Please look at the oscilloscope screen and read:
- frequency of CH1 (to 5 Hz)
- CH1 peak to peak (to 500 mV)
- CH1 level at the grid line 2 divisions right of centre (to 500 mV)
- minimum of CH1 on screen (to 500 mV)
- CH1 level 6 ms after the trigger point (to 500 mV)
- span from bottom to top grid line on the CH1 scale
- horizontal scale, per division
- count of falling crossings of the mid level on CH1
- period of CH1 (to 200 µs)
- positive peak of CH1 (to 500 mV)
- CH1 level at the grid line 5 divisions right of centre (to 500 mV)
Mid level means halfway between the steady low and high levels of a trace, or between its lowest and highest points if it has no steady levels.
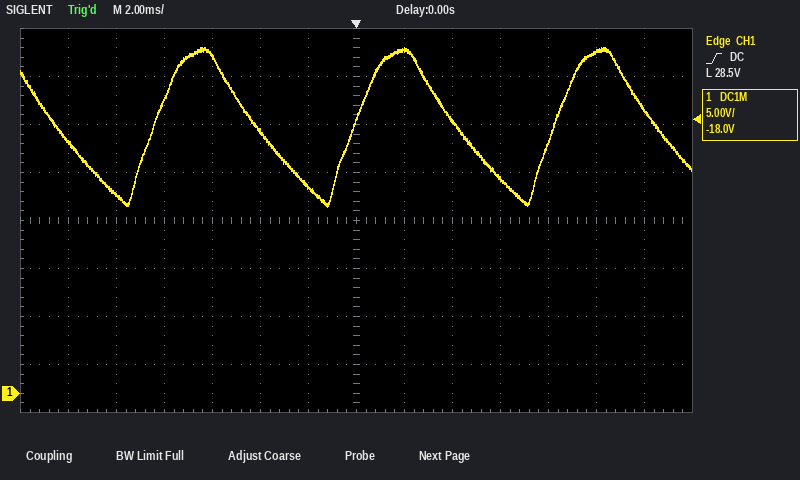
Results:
120 Hz
16.5 V
28.5 V
19.5 V
22.5 V
40 V
2 ms
4
8.4 ms
36.0 V
35.5 V
